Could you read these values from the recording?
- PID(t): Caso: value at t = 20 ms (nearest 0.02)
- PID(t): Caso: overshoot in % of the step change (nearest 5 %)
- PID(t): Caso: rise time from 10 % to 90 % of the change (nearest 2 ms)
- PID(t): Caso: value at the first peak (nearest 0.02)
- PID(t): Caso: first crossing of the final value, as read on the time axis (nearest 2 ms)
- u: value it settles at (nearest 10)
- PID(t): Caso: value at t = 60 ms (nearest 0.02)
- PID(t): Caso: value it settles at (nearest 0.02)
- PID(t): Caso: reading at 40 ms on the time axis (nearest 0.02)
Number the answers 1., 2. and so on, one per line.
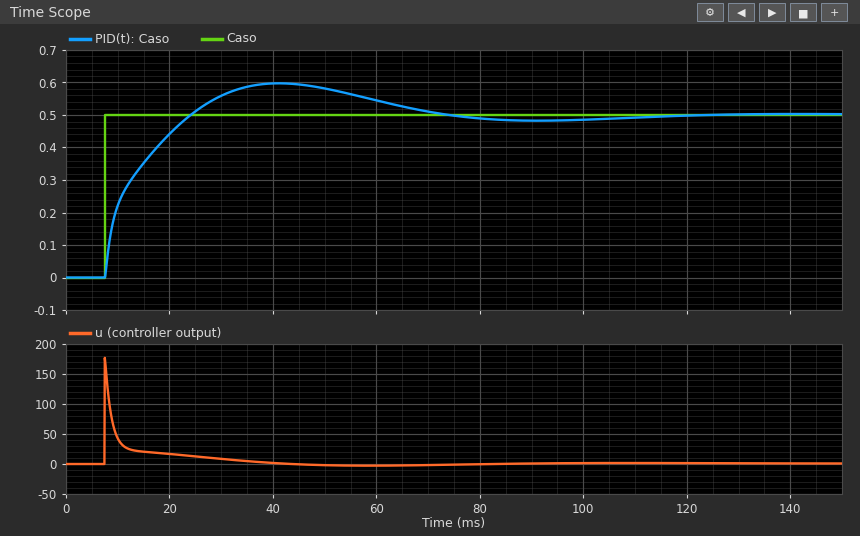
1. 0.44
2. 20 %
3. 12 ms
4. 0.60
5. 24 ms
6. 0
7. 0.54
8. 0.50
9. 0.60
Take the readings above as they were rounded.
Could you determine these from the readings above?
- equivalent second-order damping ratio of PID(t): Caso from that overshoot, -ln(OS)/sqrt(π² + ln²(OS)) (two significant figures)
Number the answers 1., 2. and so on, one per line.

1. 0.46
